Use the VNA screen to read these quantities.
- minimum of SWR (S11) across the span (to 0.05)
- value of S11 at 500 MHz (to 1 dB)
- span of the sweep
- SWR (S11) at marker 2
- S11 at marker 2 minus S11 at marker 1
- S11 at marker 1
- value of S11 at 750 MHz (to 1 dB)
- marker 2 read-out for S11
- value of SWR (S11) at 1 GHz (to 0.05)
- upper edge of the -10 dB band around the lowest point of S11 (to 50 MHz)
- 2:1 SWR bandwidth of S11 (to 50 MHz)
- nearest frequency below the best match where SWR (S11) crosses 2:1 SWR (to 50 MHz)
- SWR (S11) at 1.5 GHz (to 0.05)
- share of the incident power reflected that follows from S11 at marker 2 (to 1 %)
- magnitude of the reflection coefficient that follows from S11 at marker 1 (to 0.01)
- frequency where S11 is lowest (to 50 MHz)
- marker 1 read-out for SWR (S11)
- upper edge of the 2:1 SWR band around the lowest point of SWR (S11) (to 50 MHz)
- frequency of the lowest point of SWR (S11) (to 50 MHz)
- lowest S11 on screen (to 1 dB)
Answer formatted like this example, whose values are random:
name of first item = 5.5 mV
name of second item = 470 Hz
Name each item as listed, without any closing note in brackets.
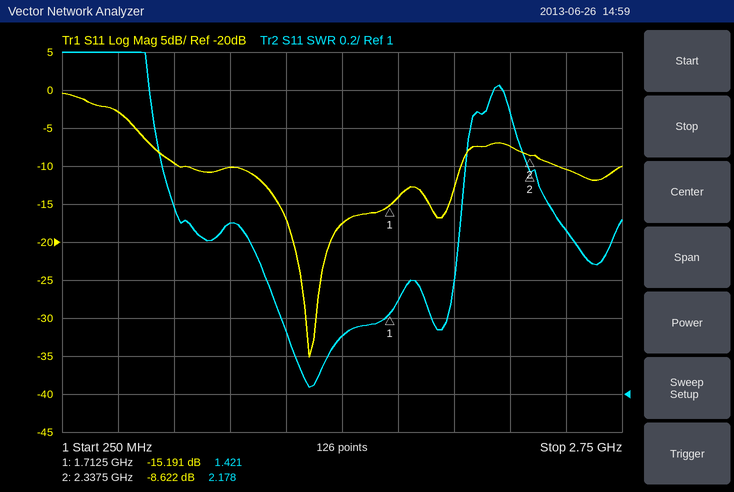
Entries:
minimum of SWR (S11) across the span = 1.05
value of S11 at 500 MHz = -3 dB
span of the sweep = 2.5 GHz
SWR (S11) at marker 2 = 2.178
S11 at marker 2 minus S11 at marker 1 = 6.569 dB
S11 at marker 1 = -15.191 dB
value of S11 at 750 MHz = -10 dB
marker 2 read-out for S11 = -8.622 dB
value of SWR (S11) at 1 GHz = 1.90
upper edge of the -10 dB band around the lowest point of S11 = 2.05 GHz
2:1 SWR bandwidth of S11 = 1.30 GHz
nearest frequency below the best match where SWR (S11) crosses 2:1 SWR = 750 MHz
SWR (S11) at 1.5 GHz = 1.30
share of the incident power reflected that follows from S11 at marker 2 = 14 %
magnitude of the reflection coefficient that follows from S11 at marker 1 = 0.17
frequency where S11 is lowest = 1.35 GHz
marker 1 read-out for SWR = 1.421
upper edge of the 2:1 SWR band around the lowest point of SWR (S11) = 2.05 GHz
frequency of the lowest point of SWR (S11) = 1.35 GHz
lowest S11 on screen = -35 dB
